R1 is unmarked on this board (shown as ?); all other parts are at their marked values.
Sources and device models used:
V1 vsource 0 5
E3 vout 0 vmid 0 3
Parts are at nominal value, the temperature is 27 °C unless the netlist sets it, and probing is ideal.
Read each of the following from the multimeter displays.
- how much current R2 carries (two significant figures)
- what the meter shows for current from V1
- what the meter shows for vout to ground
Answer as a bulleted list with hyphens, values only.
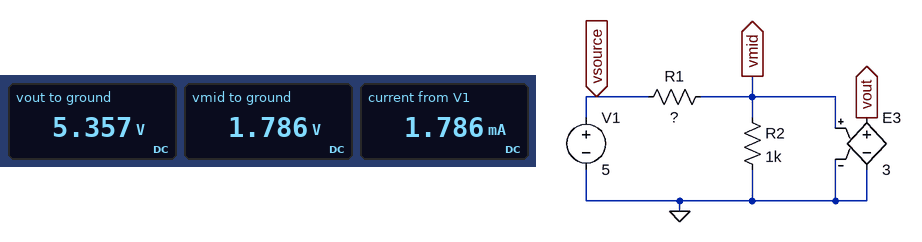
- 1.8 mA
- 1.786 mA
- 5.357 V
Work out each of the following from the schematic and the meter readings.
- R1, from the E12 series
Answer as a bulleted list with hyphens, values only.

- 1.8 kΩ
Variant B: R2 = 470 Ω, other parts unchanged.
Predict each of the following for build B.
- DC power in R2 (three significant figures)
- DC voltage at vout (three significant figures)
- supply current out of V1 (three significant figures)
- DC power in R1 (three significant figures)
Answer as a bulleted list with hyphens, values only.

- 2.28 mW
- 3.11 V
- 2.20 mA
- 8.73 mW
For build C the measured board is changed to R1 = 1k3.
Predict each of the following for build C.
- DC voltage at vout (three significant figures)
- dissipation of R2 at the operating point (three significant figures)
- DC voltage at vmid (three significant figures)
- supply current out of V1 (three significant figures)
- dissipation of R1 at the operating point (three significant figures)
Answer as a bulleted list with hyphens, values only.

- 6.52 V
- 4.73 mW
- 2.17 V
- 2.17 mA
- 6.14 mW
